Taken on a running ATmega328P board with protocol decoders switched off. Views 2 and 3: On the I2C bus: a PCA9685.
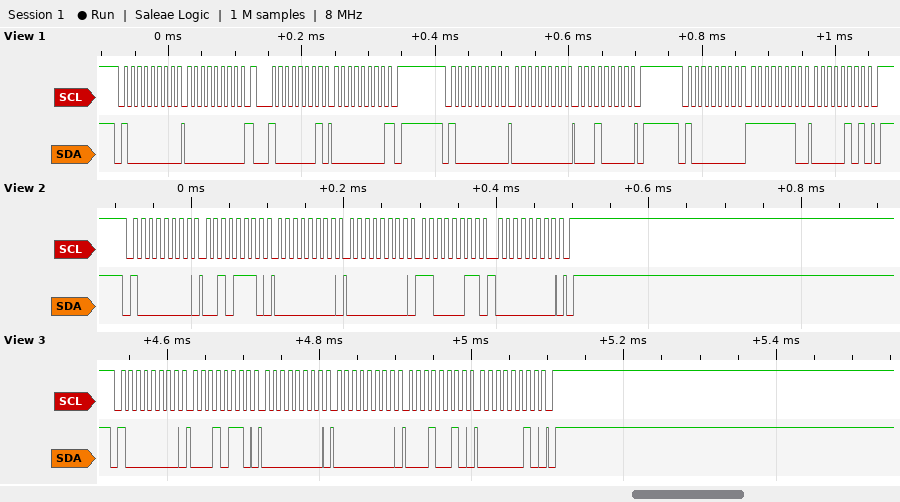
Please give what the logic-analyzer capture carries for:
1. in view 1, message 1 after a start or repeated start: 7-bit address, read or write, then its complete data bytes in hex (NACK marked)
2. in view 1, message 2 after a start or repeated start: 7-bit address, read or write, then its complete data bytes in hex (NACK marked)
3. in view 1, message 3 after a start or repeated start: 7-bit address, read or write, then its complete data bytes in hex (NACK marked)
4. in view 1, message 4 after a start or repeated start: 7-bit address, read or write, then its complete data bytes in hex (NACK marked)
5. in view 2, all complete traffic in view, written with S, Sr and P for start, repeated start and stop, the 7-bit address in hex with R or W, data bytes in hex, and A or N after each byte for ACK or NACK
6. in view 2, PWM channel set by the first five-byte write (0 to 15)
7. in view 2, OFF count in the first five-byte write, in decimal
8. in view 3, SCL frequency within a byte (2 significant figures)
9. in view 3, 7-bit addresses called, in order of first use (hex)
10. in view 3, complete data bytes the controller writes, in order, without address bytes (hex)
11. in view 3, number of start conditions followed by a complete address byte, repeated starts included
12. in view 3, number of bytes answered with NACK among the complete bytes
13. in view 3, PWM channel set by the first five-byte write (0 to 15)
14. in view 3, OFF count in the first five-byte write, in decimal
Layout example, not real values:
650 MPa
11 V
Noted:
0x40 write: 00
0x40 read: 00 NACK
0x40 write: 00 10
0x40 write: FE 05
S 40W A 2E A 00 A 00 A C3 A 00 A P
10
195
100 kHz
0x40
16 00 00 12 02
1
0
4
530
